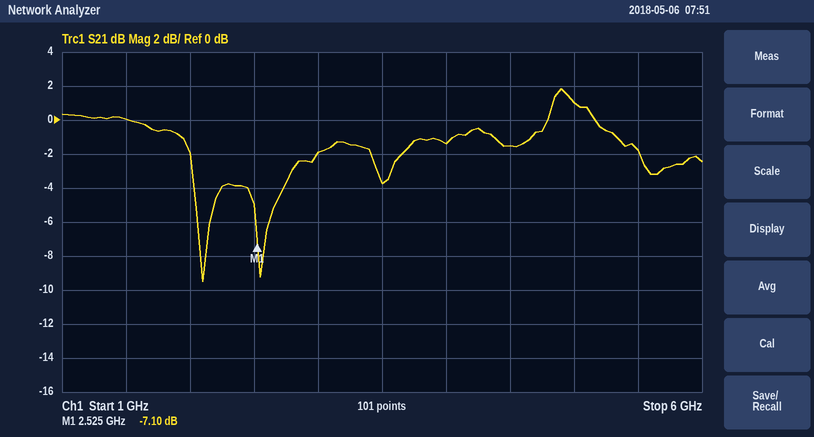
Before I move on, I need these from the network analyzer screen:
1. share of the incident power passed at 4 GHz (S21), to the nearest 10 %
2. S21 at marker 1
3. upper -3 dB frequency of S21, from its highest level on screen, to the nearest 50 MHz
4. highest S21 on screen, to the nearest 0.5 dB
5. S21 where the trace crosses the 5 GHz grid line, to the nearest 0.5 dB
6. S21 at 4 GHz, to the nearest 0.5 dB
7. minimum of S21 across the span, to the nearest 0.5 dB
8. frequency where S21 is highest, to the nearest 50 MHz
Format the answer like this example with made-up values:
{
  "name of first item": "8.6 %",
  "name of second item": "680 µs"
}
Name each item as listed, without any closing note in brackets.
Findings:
{
  "share of the incident power passed at 4 GHz (S21), to the nearest 10 %": "70 %",
  "S21 at marker 1": "-7.10 dB",
  "upper -3 dB frequency of S21, from its highest level on screen, to the nearest 50 MHz": "5.35 GHz",
  "highest S21 on screen, to the nearest 0.5 dB": "2.0 dB",
  "S21 where the trace crosses the 5 GHz grid line, to the nearest 0.5 dB": "1.0 dB",
  "S21 at 4 GHz, to the nearest 0.5 dB": "-1.5 dB",
  "minimum of S21 across the span, to the nearest 0.5 dB": "-9.5 dB",
  "frequency where S21 is highest, to the nearest 50 MHz": "4.90 GHz"
}
